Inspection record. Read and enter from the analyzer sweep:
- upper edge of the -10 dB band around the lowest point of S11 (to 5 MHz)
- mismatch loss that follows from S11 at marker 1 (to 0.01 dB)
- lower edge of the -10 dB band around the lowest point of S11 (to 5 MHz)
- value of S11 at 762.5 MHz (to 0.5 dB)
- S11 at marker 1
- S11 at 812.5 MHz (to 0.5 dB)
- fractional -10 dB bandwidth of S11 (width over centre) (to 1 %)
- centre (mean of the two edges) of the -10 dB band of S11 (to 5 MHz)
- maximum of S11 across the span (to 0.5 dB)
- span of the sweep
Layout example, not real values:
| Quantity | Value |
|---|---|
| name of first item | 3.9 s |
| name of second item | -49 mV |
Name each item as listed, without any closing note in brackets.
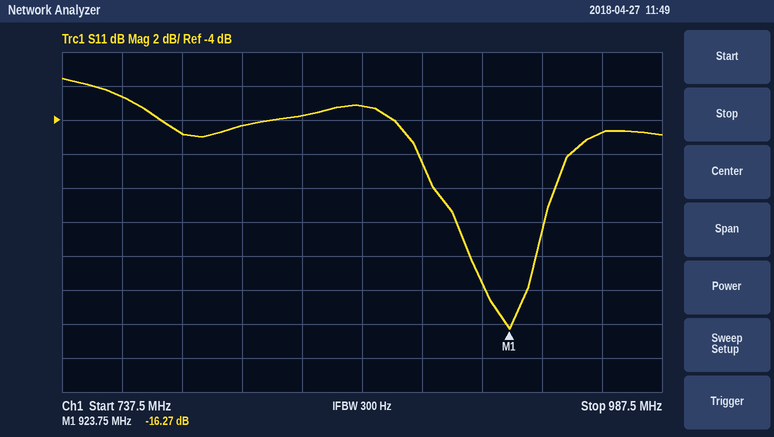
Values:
| Quantity | Value |
|---|---|
| upper edge of the -10 dB band around the lowest point of S11 | 940 MHz |
| mismatch loss that follows from S11 at marker 1 | 0.10 dB |
| lower edge of the -10 dB band around the lowest point of S11 | 900 MHz |
| value of S11 at 762.5 MHz | -2.5 dB |
| S11 at marker 1 | -16.27 dB |
| S11 at 812.5 MHz | -4.5 dB |
| fractional -10 dB bandwidth of S11 (width over centre) | 4 % |
| centre (mean of the two edges) of the -10 dB band of S11 | 920 MHz |
| maximum of S11 across the span | -1.5 dB |
| span of the sweep | 250 MHz |
